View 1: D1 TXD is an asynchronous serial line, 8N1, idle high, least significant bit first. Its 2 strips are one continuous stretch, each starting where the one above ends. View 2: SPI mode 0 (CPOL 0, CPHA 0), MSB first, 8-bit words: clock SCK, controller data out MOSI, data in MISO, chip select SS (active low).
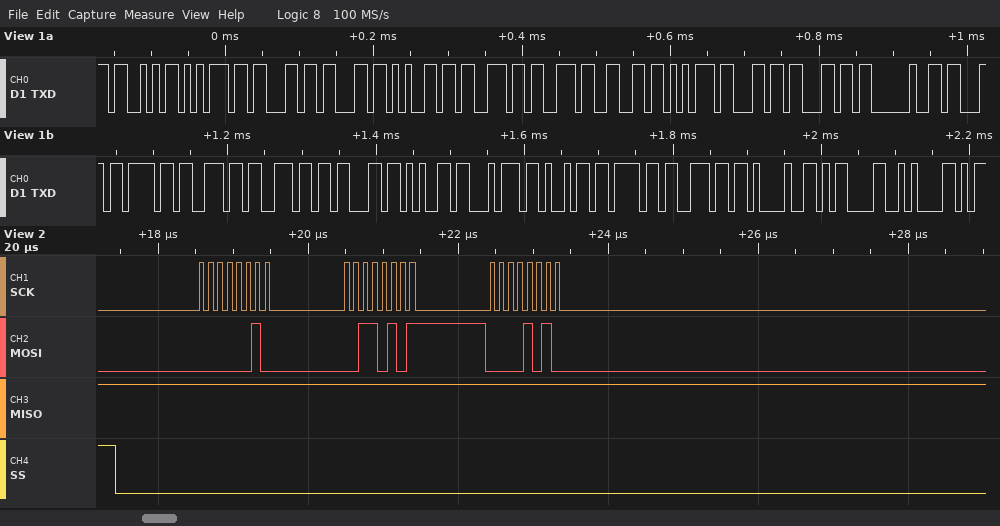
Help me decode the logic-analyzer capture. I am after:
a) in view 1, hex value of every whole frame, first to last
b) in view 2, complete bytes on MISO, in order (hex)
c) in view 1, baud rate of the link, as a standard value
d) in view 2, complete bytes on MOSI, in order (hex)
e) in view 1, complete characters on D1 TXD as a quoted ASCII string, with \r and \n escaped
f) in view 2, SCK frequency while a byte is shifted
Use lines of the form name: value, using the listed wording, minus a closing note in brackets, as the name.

in view 1, hex value of every whole frame, first to last: 53 75 63 63 65 73 73 66 75 6C 6C 20 63 6F 6E 6E 63 65 74 69 6F 6E 21 0D 0A
in view 2, complete bytes on MISO, in order: FF FF FF
in view 1, baud rate of the link, as a standard value: 115200 baud
in view 2, complete bytes on MOSI, in order: 02 35 0A
in view 1, complete characters on D1 TXD as a quoted ASCII string, with \r and \n escaped: "Successfull conncetion!\r\n"
in view 2, SCK frequency while a byte is shifted: 8 MHz
